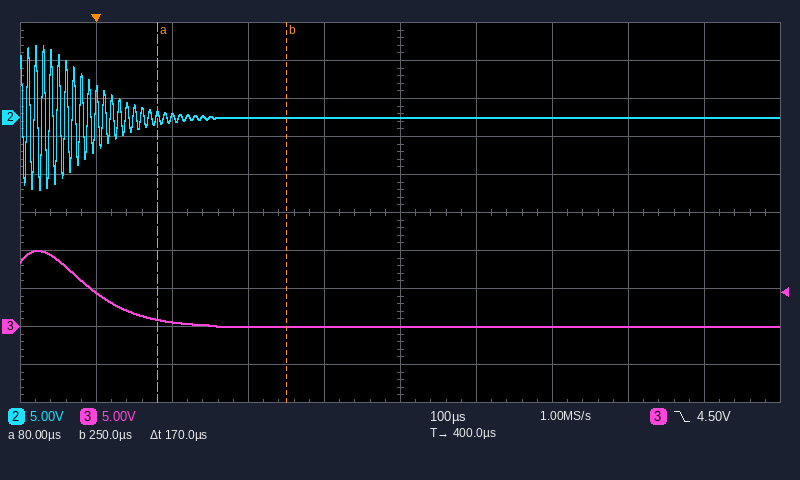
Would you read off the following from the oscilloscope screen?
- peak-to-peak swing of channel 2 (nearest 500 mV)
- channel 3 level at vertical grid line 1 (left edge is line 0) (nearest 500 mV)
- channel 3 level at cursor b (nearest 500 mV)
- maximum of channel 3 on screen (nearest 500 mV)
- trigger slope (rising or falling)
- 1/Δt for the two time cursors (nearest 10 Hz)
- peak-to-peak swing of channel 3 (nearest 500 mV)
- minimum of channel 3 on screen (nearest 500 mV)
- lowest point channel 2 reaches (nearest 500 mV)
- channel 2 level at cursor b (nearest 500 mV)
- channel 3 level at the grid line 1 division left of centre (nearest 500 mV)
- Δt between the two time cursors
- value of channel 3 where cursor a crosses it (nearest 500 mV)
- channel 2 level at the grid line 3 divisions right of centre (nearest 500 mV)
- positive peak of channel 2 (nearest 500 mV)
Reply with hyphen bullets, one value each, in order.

- 19.0 V
- 4.5 V
- 0.0 V
- 10.0 V
- falling
- 5.88 kHz
- 10.0 V
- 0.0 V
- -9.5 V
- 0.0 V
- 0.0 V
- 170 µs
- 1.0 V
- 0.0 V
- 9.5 V
